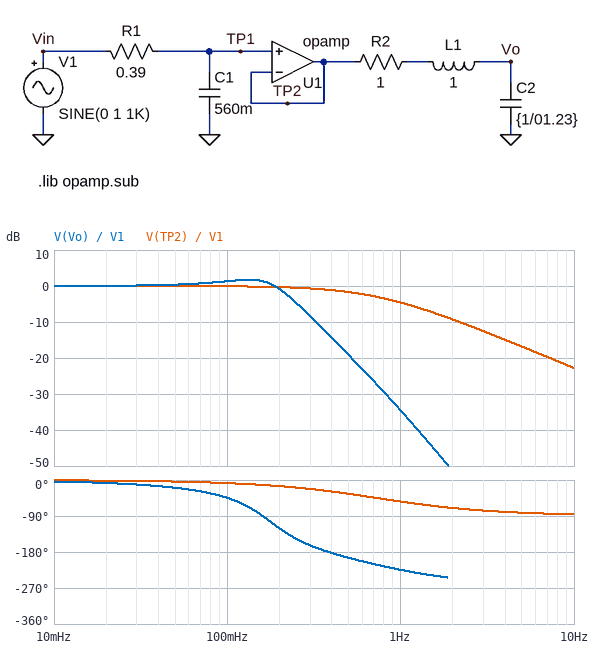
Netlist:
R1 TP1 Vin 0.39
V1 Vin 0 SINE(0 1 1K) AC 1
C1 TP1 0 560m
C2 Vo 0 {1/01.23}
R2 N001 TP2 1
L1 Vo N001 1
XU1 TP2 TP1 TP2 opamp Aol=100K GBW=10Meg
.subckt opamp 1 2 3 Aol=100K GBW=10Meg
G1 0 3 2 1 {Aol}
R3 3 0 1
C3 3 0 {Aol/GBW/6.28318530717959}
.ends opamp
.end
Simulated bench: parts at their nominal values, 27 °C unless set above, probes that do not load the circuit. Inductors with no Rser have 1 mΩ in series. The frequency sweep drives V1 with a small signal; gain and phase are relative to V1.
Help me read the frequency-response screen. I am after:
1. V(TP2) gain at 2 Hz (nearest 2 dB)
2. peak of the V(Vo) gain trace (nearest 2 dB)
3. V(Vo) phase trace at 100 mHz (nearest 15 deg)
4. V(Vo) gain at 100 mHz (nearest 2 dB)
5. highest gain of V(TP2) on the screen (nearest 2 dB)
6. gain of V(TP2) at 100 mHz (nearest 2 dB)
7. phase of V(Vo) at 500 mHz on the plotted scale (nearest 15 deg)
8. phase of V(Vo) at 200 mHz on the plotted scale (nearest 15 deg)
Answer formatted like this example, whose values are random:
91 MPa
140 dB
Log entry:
-10 dB
2 dB
-45 deg
2 dB
0 dB
0 dB
-195 deg
-120 deg
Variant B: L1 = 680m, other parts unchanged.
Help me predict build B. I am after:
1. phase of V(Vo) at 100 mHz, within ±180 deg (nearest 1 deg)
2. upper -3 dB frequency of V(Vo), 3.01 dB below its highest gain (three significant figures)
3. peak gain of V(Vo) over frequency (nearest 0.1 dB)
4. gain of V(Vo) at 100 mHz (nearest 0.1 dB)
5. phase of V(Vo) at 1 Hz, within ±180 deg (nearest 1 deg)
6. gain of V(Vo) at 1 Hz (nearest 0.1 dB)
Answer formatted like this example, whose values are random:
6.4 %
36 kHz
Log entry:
-41 deg
240 mHz
0.6 dB
0.5 dB
140 deg
-31.2 dB
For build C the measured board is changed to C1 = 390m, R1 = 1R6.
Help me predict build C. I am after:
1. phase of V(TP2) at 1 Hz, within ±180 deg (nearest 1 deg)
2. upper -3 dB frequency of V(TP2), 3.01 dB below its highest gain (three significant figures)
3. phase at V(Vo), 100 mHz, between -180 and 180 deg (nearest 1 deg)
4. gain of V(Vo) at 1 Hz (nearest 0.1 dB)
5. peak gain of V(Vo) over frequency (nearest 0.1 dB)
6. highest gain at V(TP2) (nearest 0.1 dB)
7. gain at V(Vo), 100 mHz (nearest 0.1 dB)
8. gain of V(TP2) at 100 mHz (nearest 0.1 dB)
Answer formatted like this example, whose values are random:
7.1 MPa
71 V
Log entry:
-76 deg
255 mHz
-58 deg
-42.1 dB
0.9 dB
0 dB
0.8 dB
-0.6 dB
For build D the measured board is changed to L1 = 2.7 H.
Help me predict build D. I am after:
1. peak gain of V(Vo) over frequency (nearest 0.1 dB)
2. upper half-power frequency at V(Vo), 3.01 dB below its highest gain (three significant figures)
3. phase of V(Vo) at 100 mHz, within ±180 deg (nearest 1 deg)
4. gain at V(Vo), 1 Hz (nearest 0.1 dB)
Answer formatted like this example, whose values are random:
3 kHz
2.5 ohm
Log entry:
5.5 dB
126 mHz
-83 deg
-43.3 dB
